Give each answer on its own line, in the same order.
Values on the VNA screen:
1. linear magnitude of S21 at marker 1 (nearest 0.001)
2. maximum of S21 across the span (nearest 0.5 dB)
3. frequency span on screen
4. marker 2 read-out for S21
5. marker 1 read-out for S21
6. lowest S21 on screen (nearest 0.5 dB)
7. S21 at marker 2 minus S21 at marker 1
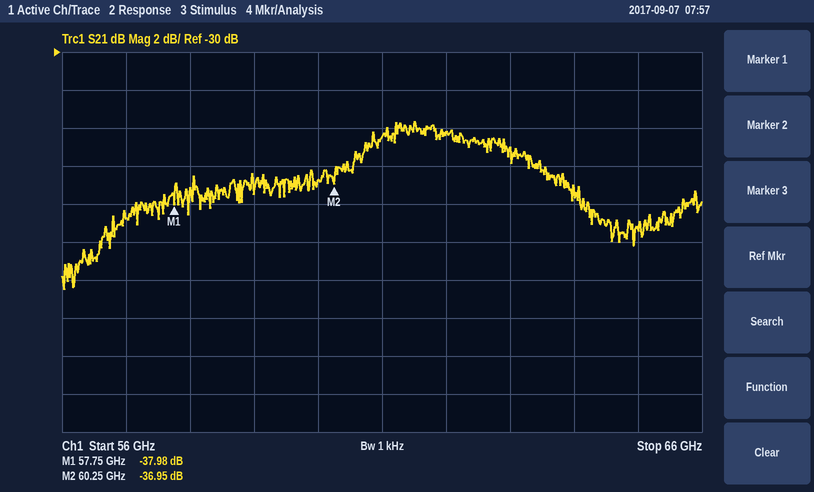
0.013
-33.5 dB
10 GHz
-36.95 dB
-37.98 dB
-42.5 dB
1.03 dB
